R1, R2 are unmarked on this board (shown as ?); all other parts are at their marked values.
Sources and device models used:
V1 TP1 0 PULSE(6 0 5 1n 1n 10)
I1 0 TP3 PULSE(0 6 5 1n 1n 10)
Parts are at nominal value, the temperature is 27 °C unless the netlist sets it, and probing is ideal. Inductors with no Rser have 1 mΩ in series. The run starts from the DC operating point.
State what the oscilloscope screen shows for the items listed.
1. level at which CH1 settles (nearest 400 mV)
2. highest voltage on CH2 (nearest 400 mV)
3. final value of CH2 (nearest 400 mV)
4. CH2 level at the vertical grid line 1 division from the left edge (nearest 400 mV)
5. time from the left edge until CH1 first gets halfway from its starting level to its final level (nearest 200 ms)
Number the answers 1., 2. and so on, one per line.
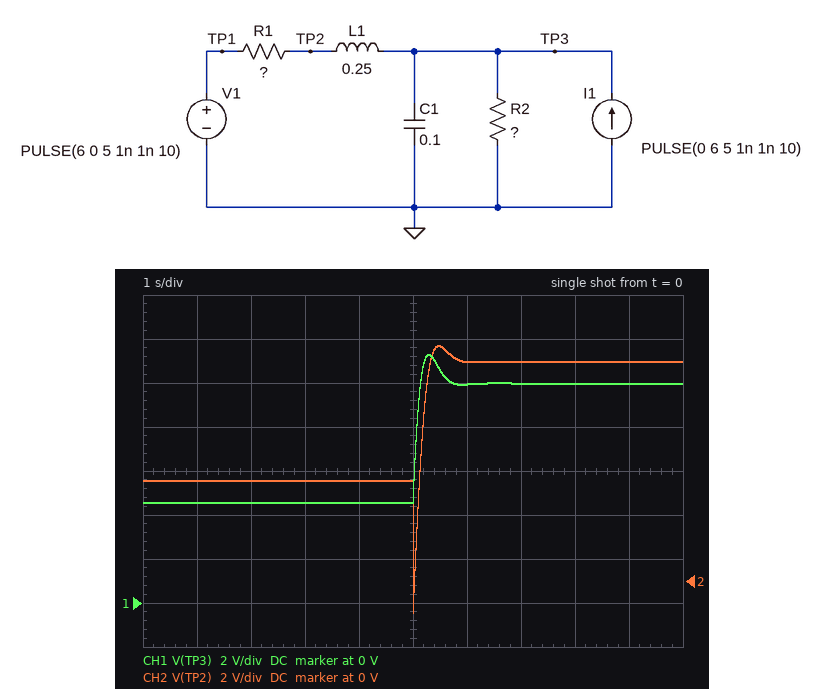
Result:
1. 10.0 V
2. 10.8 V
3. 10.0 V
4. 4.4 V
5. 5.0 s
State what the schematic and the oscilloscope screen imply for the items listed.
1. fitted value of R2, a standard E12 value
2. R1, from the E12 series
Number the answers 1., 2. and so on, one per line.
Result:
1. 6.8 Ω
2. 2.2 Ω
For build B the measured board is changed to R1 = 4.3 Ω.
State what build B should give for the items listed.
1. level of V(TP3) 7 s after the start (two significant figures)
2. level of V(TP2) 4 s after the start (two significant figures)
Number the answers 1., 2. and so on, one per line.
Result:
1. 16 V
2. 3.7 V
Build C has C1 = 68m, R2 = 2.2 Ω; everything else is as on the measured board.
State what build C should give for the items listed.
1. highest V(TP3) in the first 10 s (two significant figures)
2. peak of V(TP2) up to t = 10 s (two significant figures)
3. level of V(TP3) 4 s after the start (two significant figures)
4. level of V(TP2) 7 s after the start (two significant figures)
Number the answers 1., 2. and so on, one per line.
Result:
1. 8.4 V
2. 7.1 V
3. 3.0 V
4. 6.6 V
